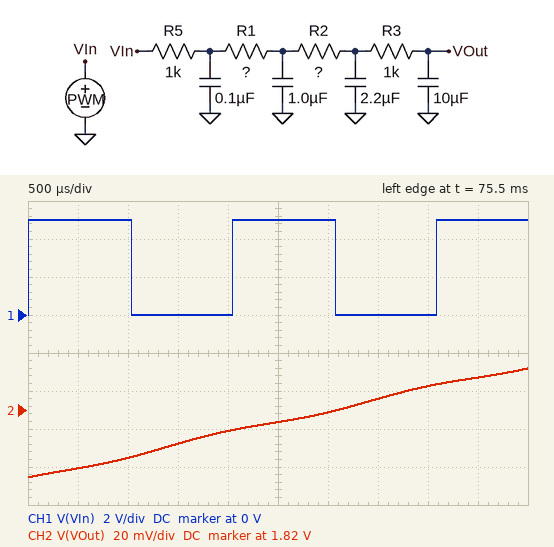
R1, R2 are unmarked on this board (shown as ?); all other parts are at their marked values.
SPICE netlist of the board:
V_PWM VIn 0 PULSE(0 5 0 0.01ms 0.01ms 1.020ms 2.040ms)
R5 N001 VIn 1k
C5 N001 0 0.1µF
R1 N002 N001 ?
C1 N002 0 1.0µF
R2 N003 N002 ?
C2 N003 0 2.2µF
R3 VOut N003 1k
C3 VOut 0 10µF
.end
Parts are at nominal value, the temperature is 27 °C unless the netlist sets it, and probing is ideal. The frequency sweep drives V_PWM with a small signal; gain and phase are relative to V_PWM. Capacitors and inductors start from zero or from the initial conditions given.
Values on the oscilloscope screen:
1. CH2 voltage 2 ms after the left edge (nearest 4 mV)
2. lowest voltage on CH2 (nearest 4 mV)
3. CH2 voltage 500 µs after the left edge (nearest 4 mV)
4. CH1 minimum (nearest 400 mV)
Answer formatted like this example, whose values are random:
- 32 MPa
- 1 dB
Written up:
- 1.808 V
- 1.784 V
- 1.788 V
- 0 V
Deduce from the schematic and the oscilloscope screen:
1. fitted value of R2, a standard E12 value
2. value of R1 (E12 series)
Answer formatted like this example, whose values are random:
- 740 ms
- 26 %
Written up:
- 2.7 kΩ
- 470 Ω
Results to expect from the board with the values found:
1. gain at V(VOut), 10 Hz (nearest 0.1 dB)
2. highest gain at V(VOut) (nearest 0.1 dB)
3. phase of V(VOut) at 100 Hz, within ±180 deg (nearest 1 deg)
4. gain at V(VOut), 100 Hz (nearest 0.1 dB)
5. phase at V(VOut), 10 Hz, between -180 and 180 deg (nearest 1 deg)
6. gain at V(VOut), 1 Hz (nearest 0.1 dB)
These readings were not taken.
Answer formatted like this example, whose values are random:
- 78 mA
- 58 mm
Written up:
- -11.9 dB
- 0 dB
- -166 deg
- -36.1 dB
- -85 deg
- -0.6 dB
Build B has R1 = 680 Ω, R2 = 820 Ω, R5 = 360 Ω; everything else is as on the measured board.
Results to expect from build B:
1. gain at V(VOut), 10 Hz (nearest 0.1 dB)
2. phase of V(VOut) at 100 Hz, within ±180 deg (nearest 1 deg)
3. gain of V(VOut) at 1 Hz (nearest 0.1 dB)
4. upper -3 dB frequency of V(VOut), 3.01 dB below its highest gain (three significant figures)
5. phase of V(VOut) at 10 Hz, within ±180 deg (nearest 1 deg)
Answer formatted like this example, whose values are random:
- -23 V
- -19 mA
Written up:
- -7.0 dB
- -146 deg
- -0.2 dB
- 4.99 Hz
- -70 deg
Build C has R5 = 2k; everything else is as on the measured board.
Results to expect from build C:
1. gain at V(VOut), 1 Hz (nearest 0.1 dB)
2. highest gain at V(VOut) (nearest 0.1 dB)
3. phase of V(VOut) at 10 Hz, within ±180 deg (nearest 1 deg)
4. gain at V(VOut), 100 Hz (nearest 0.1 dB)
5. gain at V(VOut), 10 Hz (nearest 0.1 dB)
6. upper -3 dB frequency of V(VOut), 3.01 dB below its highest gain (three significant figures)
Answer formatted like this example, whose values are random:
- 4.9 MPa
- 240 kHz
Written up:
- -0.8 dB
- 0 dB
- -89 deg
- -39.0 dB
- -13.5 dB
- 2.19 Hz
